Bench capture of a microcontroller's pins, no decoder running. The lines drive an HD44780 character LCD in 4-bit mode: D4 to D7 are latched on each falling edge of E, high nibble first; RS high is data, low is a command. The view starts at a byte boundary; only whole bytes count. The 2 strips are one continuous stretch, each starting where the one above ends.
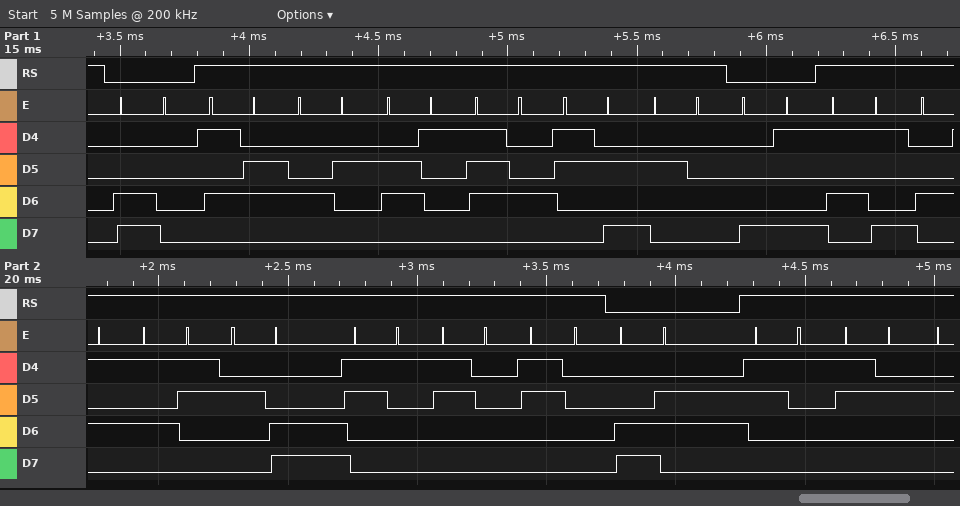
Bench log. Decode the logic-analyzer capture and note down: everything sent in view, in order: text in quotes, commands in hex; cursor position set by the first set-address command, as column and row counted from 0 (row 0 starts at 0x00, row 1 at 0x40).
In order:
0xC0 "VBat: " 0x89 "YES,100" 0xC6 "12"
column 0, row 1
